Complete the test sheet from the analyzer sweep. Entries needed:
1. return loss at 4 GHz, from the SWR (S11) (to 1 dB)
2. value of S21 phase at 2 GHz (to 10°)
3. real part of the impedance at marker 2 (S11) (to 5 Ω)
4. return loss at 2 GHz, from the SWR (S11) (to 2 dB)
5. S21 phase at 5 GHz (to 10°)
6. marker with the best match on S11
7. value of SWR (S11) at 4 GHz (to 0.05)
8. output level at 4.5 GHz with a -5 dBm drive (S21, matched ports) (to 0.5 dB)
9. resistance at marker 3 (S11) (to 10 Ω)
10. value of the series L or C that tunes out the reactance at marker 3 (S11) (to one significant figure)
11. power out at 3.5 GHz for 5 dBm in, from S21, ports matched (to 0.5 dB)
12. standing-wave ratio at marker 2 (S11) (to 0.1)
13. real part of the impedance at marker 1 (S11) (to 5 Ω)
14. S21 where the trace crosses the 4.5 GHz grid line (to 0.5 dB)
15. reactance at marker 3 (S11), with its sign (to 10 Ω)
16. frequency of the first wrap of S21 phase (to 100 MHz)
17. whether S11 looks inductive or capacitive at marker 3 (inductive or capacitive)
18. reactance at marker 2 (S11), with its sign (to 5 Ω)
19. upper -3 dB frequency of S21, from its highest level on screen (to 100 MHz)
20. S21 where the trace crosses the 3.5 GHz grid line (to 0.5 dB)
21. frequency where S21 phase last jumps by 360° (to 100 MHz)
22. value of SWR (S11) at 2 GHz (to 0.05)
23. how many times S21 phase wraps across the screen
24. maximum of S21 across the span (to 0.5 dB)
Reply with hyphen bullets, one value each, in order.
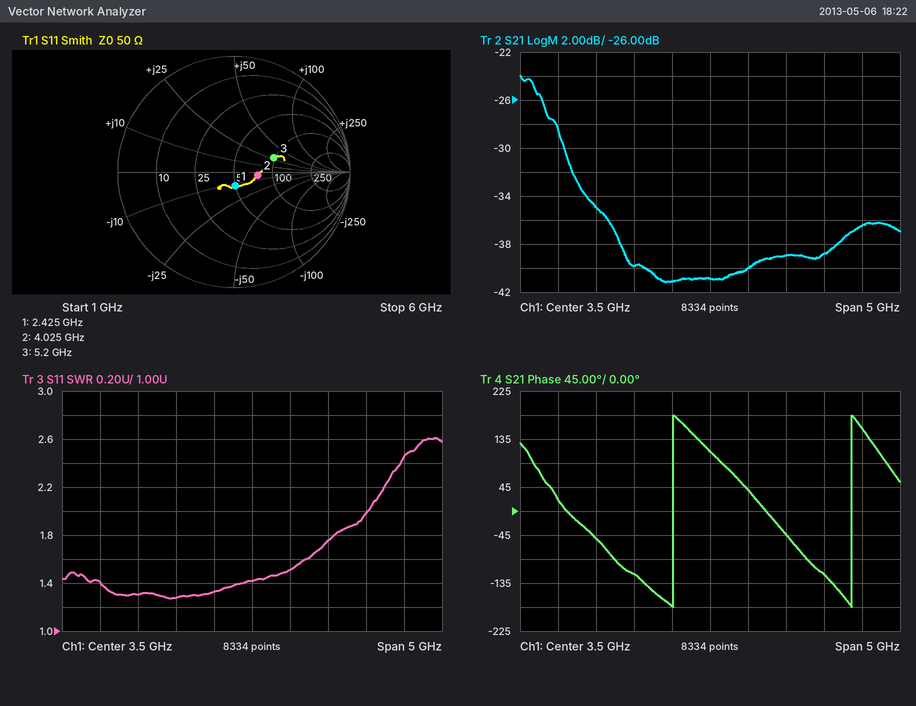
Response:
- 14 dB
- -50°
- 75 Ω
- 18 dB
- -120°
- marker 1
- 1.50
- -44.0 dBm
- 100 Ω
- 1 pF
- -36.0 dBm
- 1.5
- 50 Ω
- -39.0 dB
- +30 Ω
- 3.0 GHz
- inductive
- -5 Ω
- 1.3 GHz
- -41.0 dB
- 5.4 GHz
- 1.30
- 2
- -24.0 dB
